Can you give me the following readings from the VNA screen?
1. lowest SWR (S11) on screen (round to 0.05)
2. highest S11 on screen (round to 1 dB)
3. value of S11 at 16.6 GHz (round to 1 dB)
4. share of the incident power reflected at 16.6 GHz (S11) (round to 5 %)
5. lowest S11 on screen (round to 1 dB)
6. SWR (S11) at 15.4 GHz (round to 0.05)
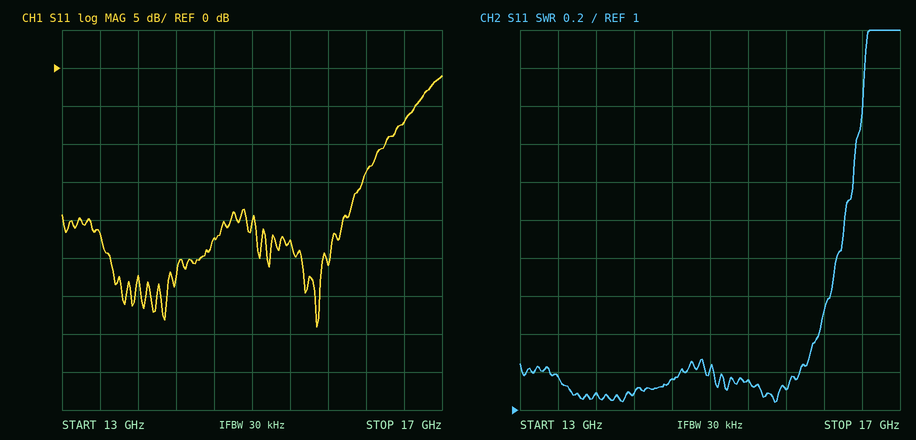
1.05
-1 dB
-7 dB
20 %
-34 dB
1.15
